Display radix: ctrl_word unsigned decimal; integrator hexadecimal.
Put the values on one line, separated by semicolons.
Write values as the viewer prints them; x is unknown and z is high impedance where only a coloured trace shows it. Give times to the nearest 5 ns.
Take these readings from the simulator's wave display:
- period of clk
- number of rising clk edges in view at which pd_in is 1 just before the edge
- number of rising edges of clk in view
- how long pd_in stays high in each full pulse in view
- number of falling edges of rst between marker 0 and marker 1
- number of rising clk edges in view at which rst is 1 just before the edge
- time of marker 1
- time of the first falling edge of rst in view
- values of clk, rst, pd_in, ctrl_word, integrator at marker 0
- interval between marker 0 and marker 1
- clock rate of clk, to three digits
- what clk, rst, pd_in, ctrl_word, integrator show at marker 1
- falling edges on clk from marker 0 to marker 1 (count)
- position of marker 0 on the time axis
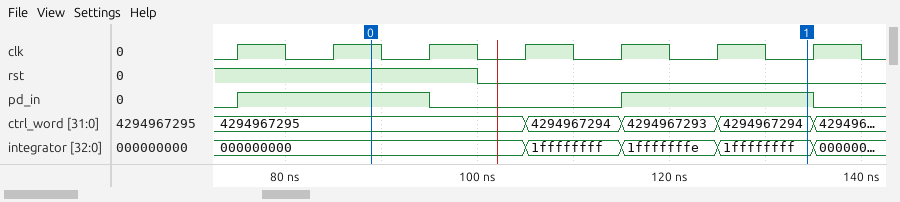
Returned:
10 ns; 4; 7; 20 ns, 20 ns; 1; 3; 135 ns; 100 ns; clk=1, rst=1, pd_in=1, ctrl_word=4294967295, integrator=000000000; 45 ns; 100 MHz; clk=0, rst=0, pd_in=1, ctrl_word=4294967294, integrator=1ffffffff; 5; 90 ns
